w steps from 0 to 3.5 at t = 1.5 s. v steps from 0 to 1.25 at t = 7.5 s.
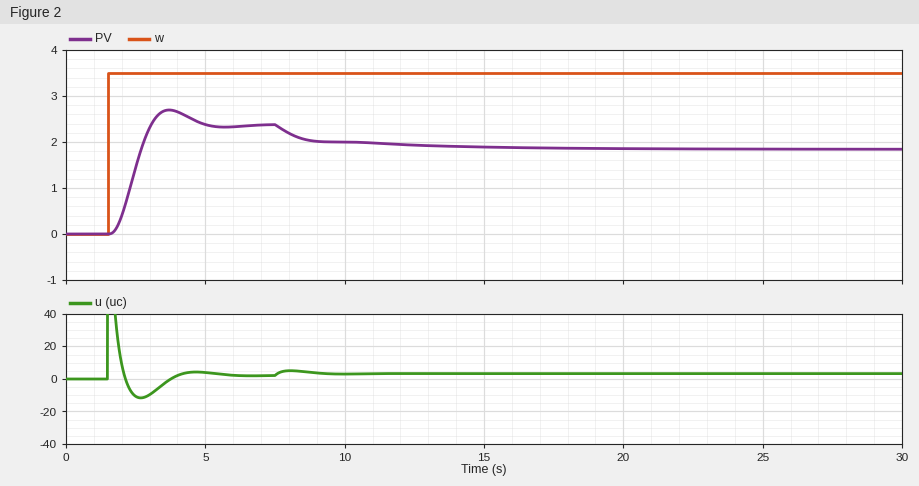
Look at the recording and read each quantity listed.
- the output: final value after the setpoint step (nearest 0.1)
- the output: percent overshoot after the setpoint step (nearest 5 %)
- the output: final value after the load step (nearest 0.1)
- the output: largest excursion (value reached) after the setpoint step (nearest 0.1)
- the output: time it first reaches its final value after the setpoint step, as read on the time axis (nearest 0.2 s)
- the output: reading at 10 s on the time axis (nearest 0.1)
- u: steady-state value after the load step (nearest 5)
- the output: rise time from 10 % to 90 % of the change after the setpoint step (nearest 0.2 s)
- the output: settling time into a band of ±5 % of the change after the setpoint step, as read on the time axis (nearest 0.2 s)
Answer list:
2.4
15 %
1.8
2.7
3.0 s
2.0
5
1.0 s
4.6 s
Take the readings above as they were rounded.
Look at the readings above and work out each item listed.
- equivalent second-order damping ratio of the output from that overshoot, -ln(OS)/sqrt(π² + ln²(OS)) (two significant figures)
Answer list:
0.52
